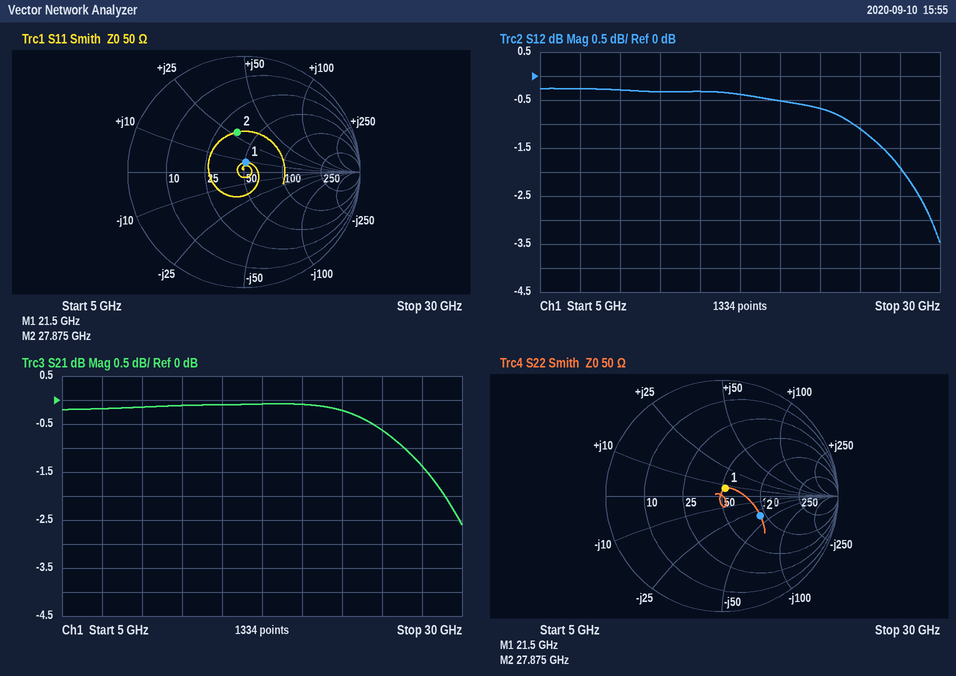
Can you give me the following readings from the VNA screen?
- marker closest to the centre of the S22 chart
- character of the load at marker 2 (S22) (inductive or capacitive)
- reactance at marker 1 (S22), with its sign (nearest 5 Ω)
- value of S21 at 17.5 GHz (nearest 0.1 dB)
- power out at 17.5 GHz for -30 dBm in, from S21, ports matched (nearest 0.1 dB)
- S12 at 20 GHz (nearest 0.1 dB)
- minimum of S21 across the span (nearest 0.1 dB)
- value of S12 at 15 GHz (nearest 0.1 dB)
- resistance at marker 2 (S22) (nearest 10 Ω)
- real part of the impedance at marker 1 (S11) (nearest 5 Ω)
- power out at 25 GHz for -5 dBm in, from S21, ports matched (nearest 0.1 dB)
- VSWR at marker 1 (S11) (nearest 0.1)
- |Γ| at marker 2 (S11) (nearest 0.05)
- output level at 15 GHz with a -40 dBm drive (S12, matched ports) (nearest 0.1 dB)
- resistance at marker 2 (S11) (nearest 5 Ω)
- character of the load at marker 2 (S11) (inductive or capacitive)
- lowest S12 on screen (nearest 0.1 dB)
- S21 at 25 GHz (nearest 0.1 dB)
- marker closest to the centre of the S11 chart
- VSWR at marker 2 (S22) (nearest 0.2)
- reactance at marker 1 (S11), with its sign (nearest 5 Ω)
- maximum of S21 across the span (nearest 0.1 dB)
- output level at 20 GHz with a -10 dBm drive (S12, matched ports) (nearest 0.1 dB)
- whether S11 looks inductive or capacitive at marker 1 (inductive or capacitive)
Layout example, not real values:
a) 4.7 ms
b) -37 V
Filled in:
a) marker 1
b) capacitive
c) +5 Ω
d) -0.1 dB
e) -30.1 dBm
f) -0.5 dB
g) -2.6 dB
h) -0.3 dB
i) 90 Ω
j) 50 Ω
k) -5.6 dBm
l) 1.2
m) 0.35
n) -40.3 dBm
o) 35 Ω
p) inductive
q) -3.5 dB
r) -0.6 dB
s) marker 1
t) 2.2
u) +10 Ω
v) -0.1 dB
w) -10.5 dBm
x) inductive
